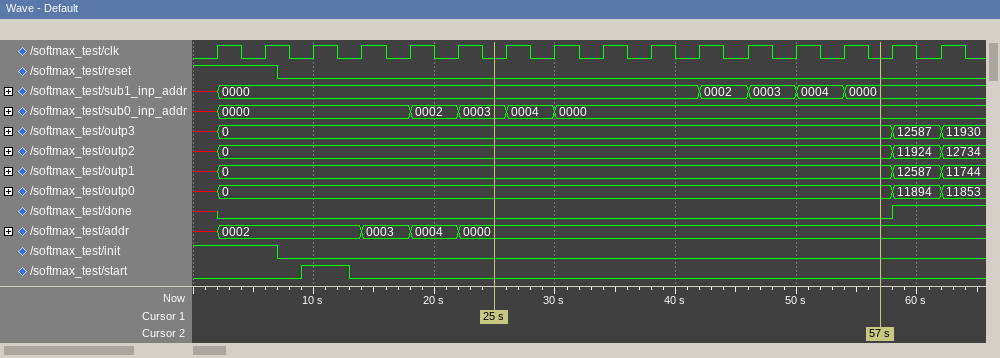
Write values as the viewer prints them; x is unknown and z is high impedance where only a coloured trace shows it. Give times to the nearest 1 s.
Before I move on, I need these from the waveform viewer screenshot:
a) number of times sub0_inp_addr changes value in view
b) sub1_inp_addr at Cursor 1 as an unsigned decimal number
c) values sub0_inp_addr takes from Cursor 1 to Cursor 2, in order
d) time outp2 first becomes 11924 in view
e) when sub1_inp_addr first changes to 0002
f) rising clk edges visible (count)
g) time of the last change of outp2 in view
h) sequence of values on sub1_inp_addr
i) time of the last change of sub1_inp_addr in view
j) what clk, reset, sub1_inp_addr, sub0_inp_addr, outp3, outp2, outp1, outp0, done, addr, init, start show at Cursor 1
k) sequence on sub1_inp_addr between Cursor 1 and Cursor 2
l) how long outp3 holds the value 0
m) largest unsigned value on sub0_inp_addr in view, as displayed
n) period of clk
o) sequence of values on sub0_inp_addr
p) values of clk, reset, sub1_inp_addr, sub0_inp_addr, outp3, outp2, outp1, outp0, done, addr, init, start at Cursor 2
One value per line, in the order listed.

5
0
0003, 0004, 0000
58 s
42 s
16
62 s
x, 0000, 0002, 0003, 0004, 0000
54 s
clk=0, reset=0, sub1_inp_addr=0000, sub0_inp_addr=0003, outp3=0, outp2=0, outp1=0, outp0=0, done=0, addr=0000, init=0, start=0
0000, 0002, 0003, 0004, 0000
56 s
0004
4 s
x, 0000, 0002, 0003, 0004, 0000
clk=0, reset=0, sub1_inp_addr=0000, sub0_inp_addr=0000, outp3=0, outp2=0, outp1=0, outp0=0, done=0, addr=0000, init=0, start=0
